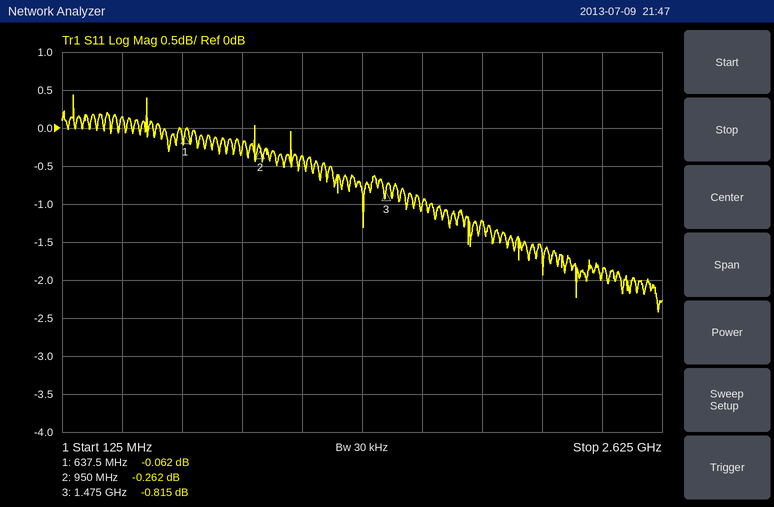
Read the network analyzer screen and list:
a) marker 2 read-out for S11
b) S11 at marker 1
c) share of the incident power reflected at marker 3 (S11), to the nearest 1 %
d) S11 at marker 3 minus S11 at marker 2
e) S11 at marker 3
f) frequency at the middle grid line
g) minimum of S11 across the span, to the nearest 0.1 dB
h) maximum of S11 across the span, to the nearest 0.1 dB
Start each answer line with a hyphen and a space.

- -0.262 dB
- -0.062 dB
- 83 %
- -0.553 dB
- -0.815 dB
- 1.375 GHz
- -2.4 dB
- 0.4 dB
